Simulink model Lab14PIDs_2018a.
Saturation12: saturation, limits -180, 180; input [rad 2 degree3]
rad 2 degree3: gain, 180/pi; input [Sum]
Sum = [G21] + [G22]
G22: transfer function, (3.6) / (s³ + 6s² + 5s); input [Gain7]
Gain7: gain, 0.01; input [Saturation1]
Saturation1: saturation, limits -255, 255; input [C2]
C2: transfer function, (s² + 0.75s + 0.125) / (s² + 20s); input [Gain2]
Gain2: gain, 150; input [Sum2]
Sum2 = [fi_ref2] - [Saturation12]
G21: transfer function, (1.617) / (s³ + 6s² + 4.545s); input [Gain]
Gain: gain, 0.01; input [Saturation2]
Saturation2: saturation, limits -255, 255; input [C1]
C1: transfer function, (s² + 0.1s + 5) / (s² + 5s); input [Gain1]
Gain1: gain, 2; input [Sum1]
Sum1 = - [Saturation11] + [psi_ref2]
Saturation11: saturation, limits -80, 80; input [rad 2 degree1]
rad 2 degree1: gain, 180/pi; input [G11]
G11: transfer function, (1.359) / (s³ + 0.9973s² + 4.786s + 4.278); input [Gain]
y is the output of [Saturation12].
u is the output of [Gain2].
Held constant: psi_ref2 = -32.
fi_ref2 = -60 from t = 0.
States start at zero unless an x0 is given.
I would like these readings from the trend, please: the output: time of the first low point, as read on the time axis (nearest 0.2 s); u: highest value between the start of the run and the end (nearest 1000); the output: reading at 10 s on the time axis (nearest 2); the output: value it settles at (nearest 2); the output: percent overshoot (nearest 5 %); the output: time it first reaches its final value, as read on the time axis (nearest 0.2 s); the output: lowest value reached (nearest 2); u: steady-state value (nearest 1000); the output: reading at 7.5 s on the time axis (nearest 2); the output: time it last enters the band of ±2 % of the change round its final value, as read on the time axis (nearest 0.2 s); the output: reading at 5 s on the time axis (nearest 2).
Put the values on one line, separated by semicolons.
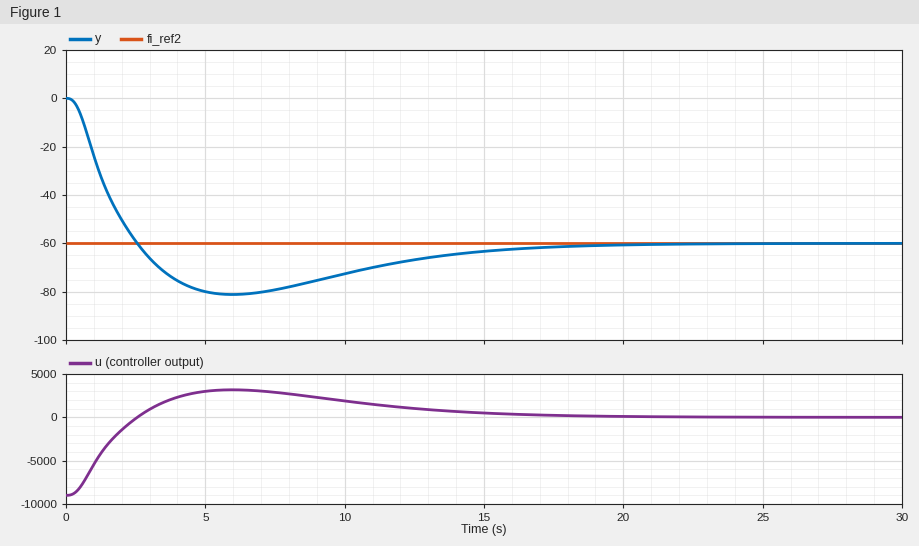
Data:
6.0 s; 3000; -72; -60; 35 %; 2.6 s; -82; 0; -80; 18.2 s; -80
